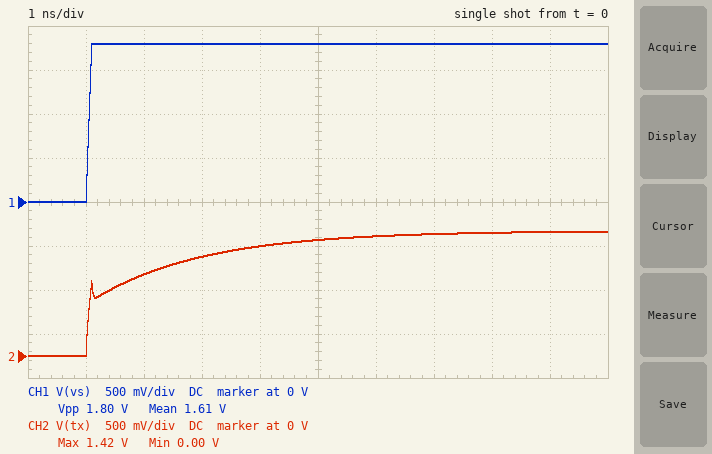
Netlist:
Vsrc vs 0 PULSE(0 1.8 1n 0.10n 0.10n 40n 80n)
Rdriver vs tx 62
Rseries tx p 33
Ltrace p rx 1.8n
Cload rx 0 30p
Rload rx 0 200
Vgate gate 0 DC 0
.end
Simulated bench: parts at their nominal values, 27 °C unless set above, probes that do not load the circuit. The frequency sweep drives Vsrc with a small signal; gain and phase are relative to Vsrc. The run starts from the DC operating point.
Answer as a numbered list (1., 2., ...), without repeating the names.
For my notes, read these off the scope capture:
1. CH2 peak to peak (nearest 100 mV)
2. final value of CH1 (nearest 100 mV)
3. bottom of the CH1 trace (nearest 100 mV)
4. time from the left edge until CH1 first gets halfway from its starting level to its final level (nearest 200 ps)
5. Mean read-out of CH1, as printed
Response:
1. 1.4 V
2. 1.8 V
3. 0 V
4. 1.0 ns
5. 1.61 V
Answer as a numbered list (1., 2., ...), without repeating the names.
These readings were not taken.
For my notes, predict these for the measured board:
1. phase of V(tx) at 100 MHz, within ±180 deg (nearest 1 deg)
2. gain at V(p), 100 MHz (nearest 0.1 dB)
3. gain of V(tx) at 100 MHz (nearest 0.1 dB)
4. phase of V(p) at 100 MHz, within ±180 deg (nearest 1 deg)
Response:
1. -22 deg
2. -7.5 dB
3. -5.0 dB
4. -51 deg
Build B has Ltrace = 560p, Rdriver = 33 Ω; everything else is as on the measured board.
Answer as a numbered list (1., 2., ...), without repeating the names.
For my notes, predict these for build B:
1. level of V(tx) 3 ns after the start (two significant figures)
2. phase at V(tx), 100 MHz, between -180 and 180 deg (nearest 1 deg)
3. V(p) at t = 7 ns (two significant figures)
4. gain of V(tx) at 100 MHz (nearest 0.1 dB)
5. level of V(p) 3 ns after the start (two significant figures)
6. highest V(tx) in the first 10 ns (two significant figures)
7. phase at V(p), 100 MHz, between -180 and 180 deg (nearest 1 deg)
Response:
1. 1.4 V
2. -15 deg
3. 1.3 V
4. -2.8 dB
5. 990 mV
6. 1.6 V
7. -43 deg
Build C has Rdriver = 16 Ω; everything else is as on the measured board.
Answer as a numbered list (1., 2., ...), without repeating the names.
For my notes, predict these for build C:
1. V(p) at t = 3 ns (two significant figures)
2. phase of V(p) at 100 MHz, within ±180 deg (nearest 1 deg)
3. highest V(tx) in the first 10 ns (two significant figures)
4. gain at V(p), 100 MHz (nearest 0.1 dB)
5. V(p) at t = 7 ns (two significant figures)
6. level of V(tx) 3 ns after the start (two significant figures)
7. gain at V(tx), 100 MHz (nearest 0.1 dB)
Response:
1. 1.2 V
2. -37 deg
3. 1.7 V
4. -3.9 dB
5. 1.4 V
6. 1.6 V
7. -1.4 dB
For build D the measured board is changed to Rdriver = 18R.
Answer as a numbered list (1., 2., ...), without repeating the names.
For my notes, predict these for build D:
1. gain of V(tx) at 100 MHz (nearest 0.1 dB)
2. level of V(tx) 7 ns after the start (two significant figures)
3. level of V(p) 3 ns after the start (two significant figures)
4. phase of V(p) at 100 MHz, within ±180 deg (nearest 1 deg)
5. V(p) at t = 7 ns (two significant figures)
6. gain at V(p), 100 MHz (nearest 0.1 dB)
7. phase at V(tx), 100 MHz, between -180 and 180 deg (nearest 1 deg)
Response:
1. -1.6 dB
2. 1.7 V
3. 1.1 V
4. -38 deg
5. 1.4 V
6. -4.1 dB
7. -9 deg
